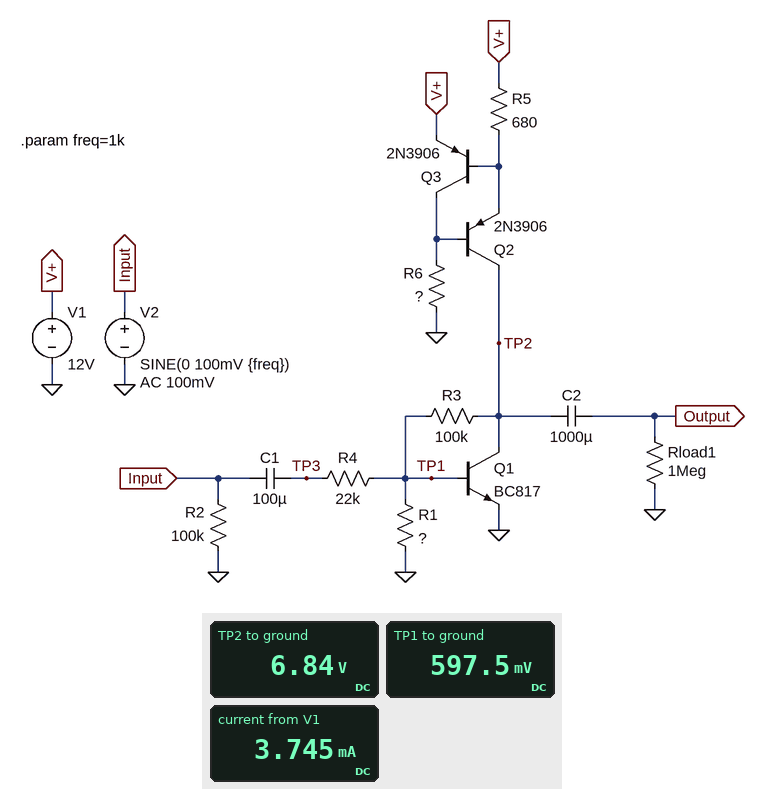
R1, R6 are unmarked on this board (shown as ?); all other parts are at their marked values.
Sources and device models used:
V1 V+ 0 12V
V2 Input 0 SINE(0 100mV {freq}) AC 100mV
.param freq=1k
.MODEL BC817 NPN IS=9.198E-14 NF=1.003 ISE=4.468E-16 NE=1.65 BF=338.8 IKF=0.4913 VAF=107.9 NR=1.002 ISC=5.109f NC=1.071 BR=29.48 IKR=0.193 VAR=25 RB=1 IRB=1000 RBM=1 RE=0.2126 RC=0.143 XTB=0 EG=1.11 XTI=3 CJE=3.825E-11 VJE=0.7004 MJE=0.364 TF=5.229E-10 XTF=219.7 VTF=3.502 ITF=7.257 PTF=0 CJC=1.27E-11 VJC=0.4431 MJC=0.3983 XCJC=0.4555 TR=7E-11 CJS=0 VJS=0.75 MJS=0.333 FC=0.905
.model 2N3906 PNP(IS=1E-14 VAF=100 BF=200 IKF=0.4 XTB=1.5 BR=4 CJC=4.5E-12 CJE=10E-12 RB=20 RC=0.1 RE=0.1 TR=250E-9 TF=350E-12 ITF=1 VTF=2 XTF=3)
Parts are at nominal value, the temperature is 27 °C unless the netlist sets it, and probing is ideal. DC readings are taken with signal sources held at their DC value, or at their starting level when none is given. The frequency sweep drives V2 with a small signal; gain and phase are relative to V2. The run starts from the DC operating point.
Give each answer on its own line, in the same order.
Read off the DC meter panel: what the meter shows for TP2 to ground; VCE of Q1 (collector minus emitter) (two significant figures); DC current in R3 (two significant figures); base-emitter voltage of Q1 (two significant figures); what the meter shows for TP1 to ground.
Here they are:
6.84 V
6.8 V
62 µA
600 mV
597.5 mV
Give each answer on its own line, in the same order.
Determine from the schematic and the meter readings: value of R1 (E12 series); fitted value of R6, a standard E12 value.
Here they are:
10 kΩ
3.9 kΩ
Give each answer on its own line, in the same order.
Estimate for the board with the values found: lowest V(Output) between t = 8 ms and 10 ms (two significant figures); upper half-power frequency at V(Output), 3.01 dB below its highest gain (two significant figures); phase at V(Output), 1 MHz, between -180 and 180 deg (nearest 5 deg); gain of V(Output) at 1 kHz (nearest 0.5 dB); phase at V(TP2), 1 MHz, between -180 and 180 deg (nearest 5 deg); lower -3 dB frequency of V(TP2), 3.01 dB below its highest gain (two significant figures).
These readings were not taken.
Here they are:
-450 mV
370 kHz
110 deg
13.0 dB
110 deg
72 mHz
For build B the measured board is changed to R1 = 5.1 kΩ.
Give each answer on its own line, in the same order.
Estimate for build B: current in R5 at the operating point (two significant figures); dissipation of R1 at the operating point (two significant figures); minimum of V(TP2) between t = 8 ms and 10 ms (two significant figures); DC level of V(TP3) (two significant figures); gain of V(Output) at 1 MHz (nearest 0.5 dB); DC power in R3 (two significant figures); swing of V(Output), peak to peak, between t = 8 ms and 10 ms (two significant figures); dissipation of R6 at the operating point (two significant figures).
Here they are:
990 µA
59 µW
11 V
550 mV
-44.0 dB
1.2 mW
4.5 mV
29 mW
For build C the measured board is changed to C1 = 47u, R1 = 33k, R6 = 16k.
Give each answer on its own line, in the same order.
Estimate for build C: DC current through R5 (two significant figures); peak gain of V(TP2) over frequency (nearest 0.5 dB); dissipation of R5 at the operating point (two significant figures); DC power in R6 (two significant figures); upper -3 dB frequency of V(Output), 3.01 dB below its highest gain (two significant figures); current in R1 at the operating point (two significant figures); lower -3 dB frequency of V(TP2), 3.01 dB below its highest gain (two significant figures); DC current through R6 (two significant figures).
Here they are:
950 µA
13.0 dB
610 µW
7.2 mW
250 kHz
18 µA
150 mHz
670 µA
